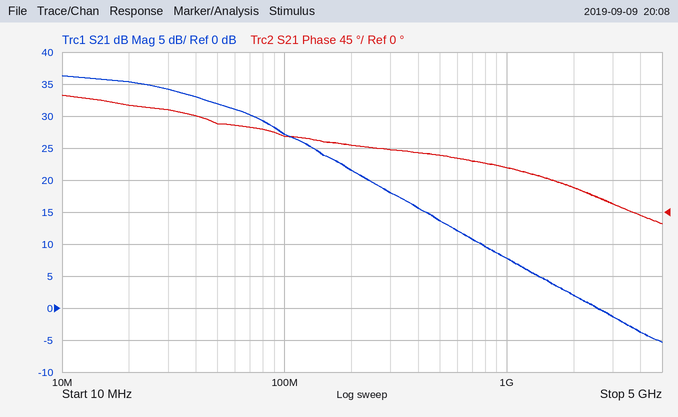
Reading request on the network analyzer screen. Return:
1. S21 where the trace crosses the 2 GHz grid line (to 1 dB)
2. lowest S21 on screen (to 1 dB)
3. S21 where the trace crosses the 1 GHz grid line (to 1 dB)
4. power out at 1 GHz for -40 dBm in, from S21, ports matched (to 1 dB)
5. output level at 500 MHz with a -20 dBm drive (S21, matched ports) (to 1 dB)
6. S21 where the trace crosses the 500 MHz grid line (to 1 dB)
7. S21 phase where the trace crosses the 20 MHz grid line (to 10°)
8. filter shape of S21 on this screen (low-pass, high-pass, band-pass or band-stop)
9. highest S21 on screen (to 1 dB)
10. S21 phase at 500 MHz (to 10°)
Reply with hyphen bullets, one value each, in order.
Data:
- 2 dB
- -5 dB
- 8 dB
- -32 dBm
- -6 dBm
- 14 dB
- 150°
- low-pass
- 36 dB
- 80°
